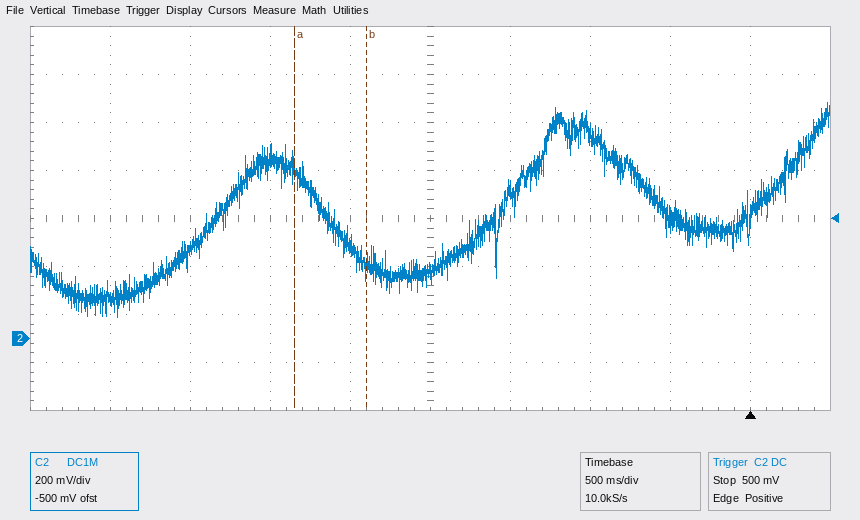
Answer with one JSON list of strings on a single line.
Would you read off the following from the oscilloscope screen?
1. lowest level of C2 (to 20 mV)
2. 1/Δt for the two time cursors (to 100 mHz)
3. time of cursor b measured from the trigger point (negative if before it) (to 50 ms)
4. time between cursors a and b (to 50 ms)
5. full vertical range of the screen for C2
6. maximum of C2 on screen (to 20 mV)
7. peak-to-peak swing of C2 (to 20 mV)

["80 mV", "2.2 Hz", "-2.40 s", "450 ms", "1.6 V", "980 mV", "900 mV"]
